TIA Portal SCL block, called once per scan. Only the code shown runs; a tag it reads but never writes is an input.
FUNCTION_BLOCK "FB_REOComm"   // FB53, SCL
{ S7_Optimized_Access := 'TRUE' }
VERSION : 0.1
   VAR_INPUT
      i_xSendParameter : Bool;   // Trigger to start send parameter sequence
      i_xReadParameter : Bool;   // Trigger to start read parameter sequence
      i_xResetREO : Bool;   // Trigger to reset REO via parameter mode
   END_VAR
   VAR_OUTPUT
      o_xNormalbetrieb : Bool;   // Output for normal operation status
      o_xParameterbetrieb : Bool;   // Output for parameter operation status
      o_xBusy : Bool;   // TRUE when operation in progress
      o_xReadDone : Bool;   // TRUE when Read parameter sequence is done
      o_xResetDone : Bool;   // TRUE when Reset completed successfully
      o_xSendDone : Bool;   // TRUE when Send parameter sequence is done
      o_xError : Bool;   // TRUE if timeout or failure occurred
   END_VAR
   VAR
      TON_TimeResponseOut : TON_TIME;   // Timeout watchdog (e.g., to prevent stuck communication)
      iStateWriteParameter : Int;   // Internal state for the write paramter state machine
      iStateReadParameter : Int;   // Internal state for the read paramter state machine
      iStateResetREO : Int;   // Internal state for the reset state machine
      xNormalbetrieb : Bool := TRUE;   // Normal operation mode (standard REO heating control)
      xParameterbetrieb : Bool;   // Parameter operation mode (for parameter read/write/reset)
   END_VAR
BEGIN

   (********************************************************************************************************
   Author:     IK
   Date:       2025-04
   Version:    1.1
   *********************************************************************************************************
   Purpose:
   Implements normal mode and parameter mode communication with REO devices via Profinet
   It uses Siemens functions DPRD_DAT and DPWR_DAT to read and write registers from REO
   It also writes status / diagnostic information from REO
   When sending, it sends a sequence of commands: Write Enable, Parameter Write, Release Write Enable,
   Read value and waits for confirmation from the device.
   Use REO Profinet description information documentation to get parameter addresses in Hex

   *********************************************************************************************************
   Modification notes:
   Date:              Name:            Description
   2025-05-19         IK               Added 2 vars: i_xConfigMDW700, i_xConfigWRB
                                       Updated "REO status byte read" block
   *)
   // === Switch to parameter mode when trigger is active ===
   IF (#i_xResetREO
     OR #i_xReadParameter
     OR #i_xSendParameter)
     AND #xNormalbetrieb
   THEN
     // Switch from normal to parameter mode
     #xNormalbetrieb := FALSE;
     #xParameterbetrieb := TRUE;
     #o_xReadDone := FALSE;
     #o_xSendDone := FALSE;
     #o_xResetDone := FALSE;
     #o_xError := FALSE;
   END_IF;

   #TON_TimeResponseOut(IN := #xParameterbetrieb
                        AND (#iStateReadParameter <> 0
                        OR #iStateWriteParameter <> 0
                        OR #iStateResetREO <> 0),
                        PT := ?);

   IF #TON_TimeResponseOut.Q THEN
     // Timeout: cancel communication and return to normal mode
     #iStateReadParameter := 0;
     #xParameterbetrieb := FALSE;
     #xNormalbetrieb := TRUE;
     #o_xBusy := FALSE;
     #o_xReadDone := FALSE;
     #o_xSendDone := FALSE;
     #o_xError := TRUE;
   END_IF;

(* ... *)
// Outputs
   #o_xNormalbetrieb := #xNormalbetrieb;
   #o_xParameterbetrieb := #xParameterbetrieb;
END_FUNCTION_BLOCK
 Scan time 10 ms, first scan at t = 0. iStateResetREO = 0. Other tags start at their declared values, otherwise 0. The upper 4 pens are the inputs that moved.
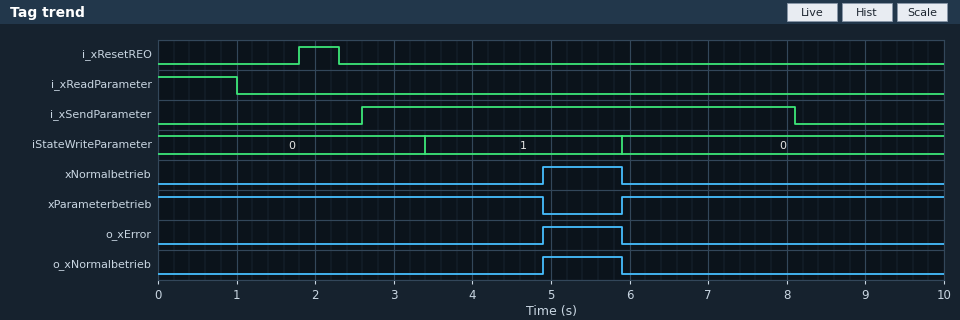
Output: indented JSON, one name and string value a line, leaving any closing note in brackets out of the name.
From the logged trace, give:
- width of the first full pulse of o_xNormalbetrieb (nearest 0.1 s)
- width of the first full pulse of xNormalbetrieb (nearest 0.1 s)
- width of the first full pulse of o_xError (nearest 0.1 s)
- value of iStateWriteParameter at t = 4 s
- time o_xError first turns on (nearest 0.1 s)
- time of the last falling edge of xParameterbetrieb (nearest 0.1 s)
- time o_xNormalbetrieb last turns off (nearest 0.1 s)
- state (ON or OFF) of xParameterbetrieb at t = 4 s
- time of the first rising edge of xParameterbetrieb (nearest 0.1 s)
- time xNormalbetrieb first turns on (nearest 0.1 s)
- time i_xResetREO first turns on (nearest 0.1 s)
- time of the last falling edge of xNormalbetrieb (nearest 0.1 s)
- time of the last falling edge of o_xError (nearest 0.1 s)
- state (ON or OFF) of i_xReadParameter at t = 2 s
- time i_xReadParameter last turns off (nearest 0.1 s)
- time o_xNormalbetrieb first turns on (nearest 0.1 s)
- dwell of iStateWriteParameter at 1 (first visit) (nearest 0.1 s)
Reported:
{
  "width of the first full pulse of o_xNormalbetrieb": "1.0 s",
  "width of the first full pulse of xNormalbetrieb": "1.0 s",
  "width of the first full pulse of o_xError": "1.0 s",
  "value of iStateWriteParameter at t = 4 s": "1",
  "time o_xError first turns on": "4.9 s",
  "time of the last falling edge of xParameterbetrieb": "4.9 s",
  "time o_xNormalbetrieb last turns off": "5.9 s",
  "state (ON or OFF) of xParameterbetrieb at t = 4 s": "ON",
  "time of the first rising edge of xParameterbetrieb": "5.9 s",
  "time xNormalbetrieb first turns on": "4.9 s",
  "time i_xResetREO first turns on": "1.8 s",
  "time of the last falling edge of xNormalbetrieb": "5.9 s",
  "time of the last falling edge of o_xError": "5.9 s",
  "state (ON or OFF) of i_xReadParameter at t = 2 s": "OFF",
  "time i_xReadParameter last turns off": "1.0 s",
  "time o_xNormalbetrieb first turns on": "4.9 s",
  "dwell of iStateWriteParameter at 1 (first visit)": "2.5 s"
}
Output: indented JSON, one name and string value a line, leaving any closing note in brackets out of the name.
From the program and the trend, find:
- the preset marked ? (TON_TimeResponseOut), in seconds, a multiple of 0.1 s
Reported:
{
  "the preset marked ? (TON_TimeResponseOut), in seconds, a multiple of 0.1 s": "1.5 s"
}
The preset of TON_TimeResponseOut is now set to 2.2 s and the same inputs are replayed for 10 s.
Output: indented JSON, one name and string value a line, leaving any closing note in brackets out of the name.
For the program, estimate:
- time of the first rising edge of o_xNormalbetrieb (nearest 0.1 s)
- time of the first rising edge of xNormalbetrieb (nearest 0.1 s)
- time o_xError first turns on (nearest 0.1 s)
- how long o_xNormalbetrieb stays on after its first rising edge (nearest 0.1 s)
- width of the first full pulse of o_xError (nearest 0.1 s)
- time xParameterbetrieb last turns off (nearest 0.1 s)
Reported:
{
  "time of the first rising edge of o_xNormalbetrieb": "5.6 s",
  "time of the first rising edge of xNormalbetrieb": "5.6 s",
  "time o_xError first turns on": "5.6 s",
  "how long o_xNormalbetrieb stays on after its first rising edge": "0.3 s",
  "width of the first full pulse of o_xError": "0.3 s",
  "time xParameterbetrieb last turns off": "5.6 s"
}
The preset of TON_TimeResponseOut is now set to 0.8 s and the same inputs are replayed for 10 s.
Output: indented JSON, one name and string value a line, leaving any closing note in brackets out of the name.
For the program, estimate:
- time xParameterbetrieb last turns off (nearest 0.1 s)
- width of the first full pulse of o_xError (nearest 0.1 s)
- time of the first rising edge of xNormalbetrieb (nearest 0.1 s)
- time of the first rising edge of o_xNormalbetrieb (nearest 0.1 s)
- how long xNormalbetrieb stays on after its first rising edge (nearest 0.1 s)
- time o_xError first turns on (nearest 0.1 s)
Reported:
{
  "time xParameterbetrieb last turns off": "4.2 s",
  "width of the first full pulse of o_xError": "1.7 s",
  "time of the first rising edge of xNormalbetrieb": "4.2 s",
  "time of the first rising edge of o_xNormalbetrieb": "4.2 s",
  "how long xNormalbetrieb stays on after its first rising edge": "1.7 s",
  "time o_xError first turns on": "4.2 s"
}
